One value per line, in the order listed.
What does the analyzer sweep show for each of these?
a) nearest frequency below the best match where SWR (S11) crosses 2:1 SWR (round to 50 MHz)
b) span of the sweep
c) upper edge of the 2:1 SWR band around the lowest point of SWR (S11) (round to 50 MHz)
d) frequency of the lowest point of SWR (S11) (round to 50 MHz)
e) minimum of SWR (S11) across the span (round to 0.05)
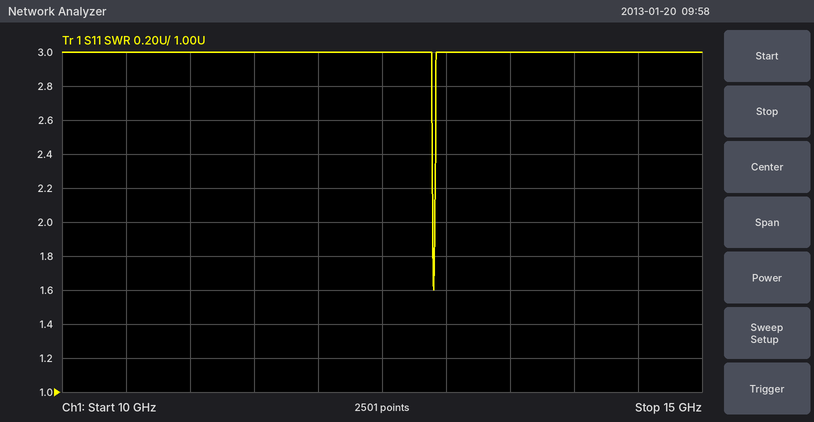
12.90 GHz
5 GHz
12.90 GHz
12.90 GHz
1.60
